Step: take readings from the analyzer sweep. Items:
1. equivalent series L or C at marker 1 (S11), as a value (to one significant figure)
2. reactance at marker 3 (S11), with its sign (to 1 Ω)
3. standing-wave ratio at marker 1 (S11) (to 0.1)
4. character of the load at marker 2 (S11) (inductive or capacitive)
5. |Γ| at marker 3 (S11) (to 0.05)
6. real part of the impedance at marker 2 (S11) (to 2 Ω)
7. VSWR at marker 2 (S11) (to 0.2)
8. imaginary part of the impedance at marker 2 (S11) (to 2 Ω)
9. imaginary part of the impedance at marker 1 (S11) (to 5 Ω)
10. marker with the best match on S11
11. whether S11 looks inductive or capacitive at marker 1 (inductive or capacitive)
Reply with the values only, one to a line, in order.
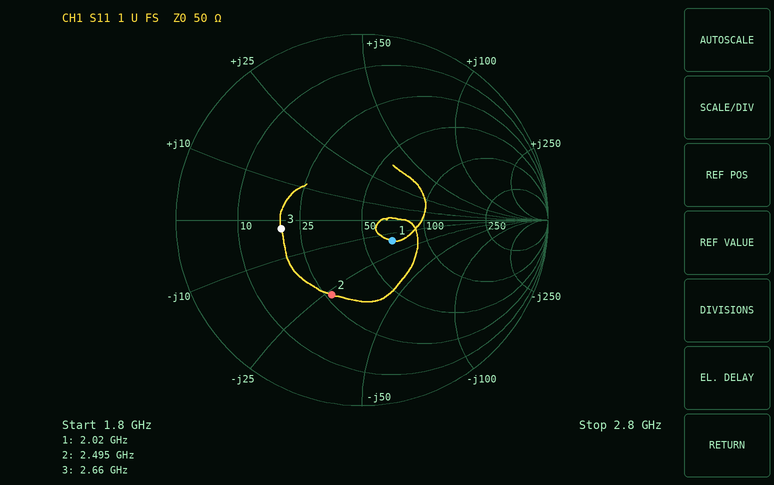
5 pF
-2 Ω
1.5
capacitive
0.45
26 Ω
2.6
-26 Ω
-15 Ω
marker 1
capacitive
